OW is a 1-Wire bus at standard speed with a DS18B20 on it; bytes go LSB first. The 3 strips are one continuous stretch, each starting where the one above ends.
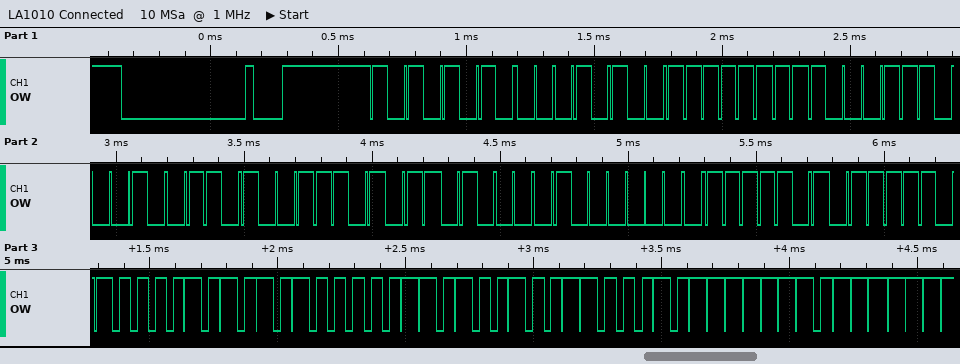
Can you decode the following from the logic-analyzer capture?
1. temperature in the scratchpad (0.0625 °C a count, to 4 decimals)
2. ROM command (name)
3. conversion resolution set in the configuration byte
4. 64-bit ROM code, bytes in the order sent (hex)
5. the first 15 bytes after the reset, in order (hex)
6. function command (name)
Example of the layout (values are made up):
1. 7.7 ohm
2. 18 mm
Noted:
1. 85.0000 °C
2. Match ROM
3. 12 bits
4. 28 FF 71 64 B9 16 02 BE
5. 55 28 FF 71 64 B9 16 02 BE BE 50 05 4B 46 7F
6. Read Scratchpad
